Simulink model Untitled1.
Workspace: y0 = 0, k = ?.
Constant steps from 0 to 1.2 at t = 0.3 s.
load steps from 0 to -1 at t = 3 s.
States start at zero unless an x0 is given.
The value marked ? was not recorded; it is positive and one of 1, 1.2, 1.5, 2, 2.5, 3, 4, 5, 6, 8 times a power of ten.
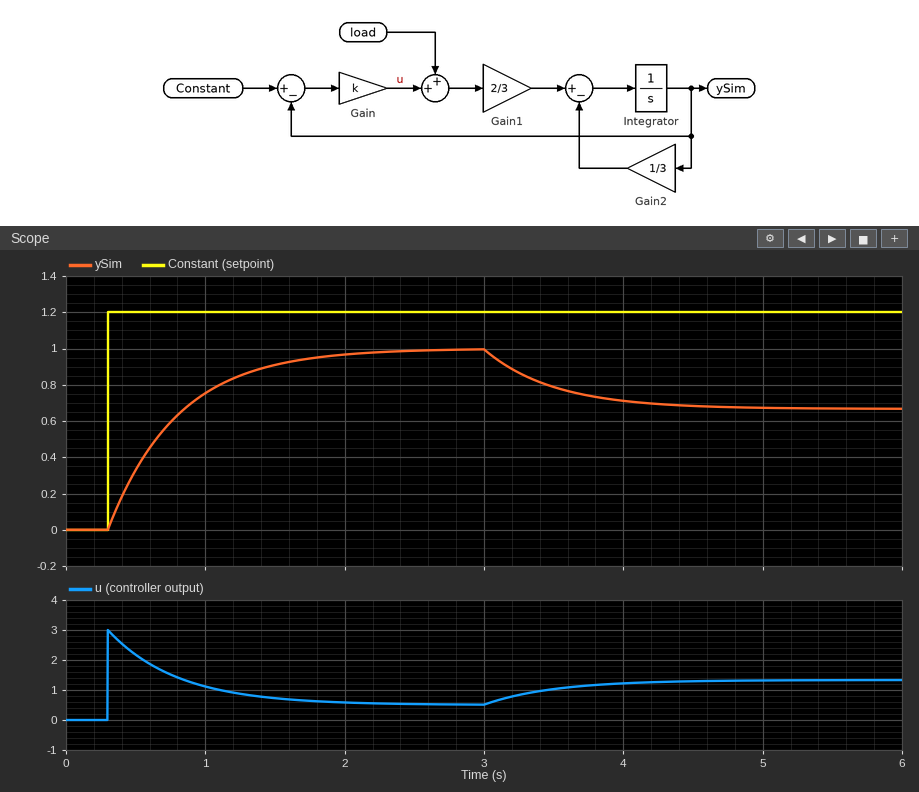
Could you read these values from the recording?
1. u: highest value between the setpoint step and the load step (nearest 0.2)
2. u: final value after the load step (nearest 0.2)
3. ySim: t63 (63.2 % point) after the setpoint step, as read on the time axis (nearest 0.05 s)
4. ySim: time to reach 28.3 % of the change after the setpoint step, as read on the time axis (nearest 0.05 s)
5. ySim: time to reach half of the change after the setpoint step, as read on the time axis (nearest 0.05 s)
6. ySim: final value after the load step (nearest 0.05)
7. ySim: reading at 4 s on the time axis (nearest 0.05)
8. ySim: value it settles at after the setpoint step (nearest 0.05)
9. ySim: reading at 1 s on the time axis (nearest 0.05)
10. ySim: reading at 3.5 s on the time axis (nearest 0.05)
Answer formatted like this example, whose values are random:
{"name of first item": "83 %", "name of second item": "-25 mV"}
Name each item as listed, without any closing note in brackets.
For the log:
{"u: highest value between the setpoint step and the load step": "3.0", "u: final value after the load step": "1.4", "ySim: t63 (63.2 % point) after the setpoint step, as read on the time axis": "0.80 s", "ySim: time to reach 28.3 % of the change after the setpoint step, as read on the time axis": "0.45 s", "ySim: time to reach half of the change after the setpoint step, as read on the time axis": "0.65 s", "ySim: final value after the load step": "0.65", "ySim: reading at 4 s on the time axis": "0.70", "ySim: value it settles at after the setpoint step": "1.00", "ySim: reading at 1 s on the time axis": "0.75", "ySim: reading at 3.5 s on the time axis": "0.80"}
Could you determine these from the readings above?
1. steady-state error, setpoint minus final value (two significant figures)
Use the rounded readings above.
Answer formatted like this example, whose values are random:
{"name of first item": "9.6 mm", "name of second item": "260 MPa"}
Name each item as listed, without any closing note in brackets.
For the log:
{"steady-state error, setpoint minus final value": "0.20"}
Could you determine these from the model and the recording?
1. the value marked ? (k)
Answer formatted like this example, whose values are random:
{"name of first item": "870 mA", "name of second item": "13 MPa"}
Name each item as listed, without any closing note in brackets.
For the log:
{"the value marked ?": "2.5"}
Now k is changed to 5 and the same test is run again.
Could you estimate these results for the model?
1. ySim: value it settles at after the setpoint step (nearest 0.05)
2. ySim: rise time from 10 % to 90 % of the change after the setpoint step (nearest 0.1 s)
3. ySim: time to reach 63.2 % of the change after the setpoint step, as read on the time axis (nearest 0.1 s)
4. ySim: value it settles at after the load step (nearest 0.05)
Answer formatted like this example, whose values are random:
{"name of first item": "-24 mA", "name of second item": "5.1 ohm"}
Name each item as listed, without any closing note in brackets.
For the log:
{"ySim: value it settles at after the setpoint step": "1.10", "ySim: rise time from 10 % to 90 % of the change after the setpoint step": "0.6 s", "ySim: time to reach 63.2 % of the change after the setpoint step, as read on the time axis": "0.6 s", "ySim: value it settles at after the load step": "0.90"}
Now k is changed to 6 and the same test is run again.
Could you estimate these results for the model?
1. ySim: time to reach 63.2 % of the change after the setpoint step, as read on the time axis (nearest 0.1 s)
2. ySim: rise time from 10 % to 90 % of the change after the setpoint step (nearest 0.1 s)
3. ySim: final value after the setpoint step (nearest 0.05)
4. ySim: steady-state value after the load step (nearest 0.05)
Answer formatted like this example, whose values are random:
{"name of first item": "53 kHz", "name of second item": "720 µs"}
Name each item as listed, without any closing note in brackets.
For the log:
{"ySim: time to reach 63.2 % of the change after the setpoint step, as read on the time axis": "0.5 s", "ySim: rise time from 10 % to 90 % of the change after the setpoint step": "0.5 s", "ySim: final value after the setpoint step": "1.10", "ySim: steady-state value after the load step": "0.95"}
